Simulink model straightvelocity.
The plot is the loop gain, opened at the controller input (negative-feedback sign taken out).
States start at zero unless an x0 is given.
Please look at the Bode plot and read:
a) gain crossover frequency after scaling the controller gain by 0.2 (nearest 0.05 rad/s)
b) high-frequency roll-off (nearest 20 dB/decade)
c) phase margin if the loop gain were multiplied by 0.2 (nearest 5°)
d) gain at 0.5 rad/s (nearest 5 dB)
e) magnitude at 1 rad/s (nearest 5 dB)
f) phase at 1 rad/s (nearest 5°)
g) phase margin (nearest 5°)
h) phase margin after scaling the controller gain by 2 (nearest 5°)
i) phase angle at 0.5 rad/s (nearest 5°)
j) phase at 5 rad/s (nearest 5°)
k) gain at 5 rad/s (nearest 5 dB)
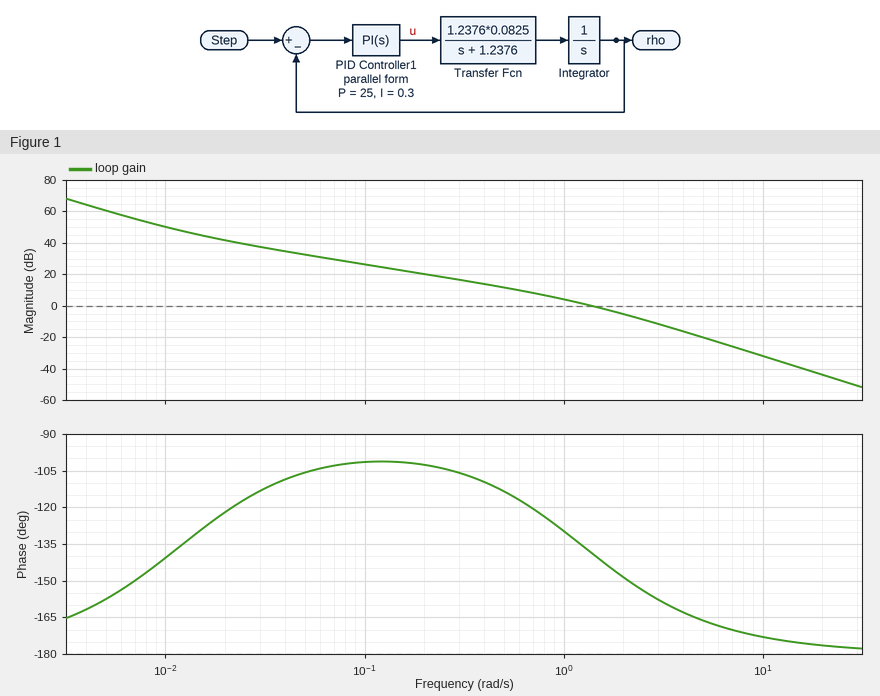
0.40 rad/s
-40 dB/decade
70°
10 dB
5 dB
-130°
40°
30°
-115°
-165°
-20 dB
